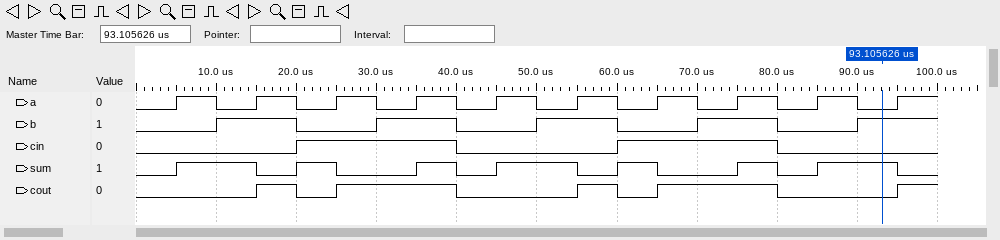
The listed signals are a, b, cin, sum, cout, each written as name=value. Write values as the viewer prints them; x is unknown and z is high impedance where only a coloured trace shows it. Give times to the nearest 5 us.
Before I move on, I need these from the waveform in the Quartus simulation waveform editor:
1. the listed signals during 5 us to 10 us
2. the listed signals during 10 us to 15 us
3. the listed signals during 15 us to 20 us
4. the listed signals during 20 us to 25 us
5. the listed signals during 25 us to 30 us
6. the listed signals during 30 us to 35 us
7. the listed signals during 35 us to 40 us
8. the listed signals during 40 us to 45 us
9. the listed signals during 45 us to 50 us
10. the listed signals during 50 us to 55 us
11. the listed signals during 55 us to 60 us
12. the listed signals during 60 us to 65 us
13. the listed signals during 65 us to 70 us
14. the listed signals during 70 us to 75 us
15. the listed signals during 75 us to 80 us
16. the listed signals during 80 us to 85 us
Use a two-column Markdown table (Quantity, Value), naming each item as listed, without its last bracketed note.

| Quantity | Value |
|---|---|
| the listed signals during 5 us to 10 us | a=1, b=0, cin=0, sum=1, cout=0 |
| the listed signals during 10 us to 15 us | a=0, b=1, cin=0, sum=1, cout=0 |
| the listed signals during 15 us to 20 us | a=1, b=1, cin=0, sum=0, cout=1 |
| the listed signals during 20 us to 25 us | a=0, b=0, cin=1, sum=1, cout=0 |
| the listed signals during 25 us to 30 us | a=1, b=0, cin=1, sum=0, cout=1 |
| the listed signals during 30 us to 35 us | a=0, b=1, cin=1, sum=0, cout=1 |
| the listed signals during 35 us to 40 us | a=1, b=1, cin=1, sum=1, cout=1 |
| the listed signals during 40 us to 45 us | a=0, b=0, cin=0, sum=0, cout=0 |
| the listed signals during 45 us to 50 us | a=1, b=0, cin=0, sum=1, cout=0 |
| the listed signals during 50 us to 55 us | a=0, b=1, cin=0, sum=1, cout=0 |
| the listed signals during 55 us to 60 us | a=1, b=1, cin=0, sum=0, cout=1 |
| the listed signals during 60 us to 65 us | a=0, b=0, cin=1, sum=1, cout=0 |
| the listed signals during 65 us to 70 us | a=1, b=0, cin=1, sum=0, cout=1 |
| the listed signals during 70 us to 75 us | a=0, b=1, cin=1, sum=0, cout=1 |
| the listed signals during 75 us to 80 us | a=1, b=1, cin=1, sum=1, cout=1 |
| the listed signals during 80 us to 85 us | a=0, b=0, cin=0, sum=0, cout=0 |
